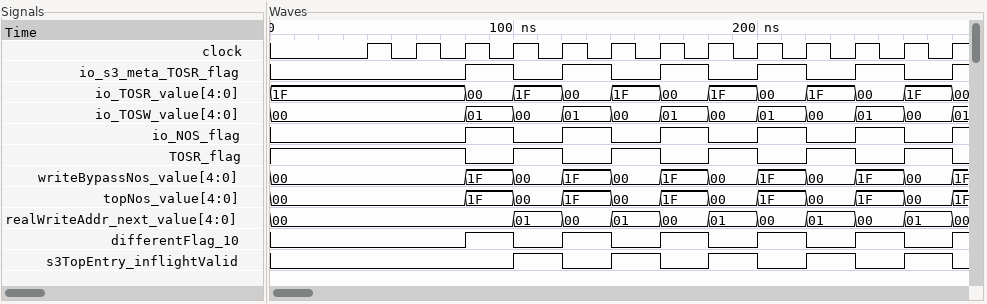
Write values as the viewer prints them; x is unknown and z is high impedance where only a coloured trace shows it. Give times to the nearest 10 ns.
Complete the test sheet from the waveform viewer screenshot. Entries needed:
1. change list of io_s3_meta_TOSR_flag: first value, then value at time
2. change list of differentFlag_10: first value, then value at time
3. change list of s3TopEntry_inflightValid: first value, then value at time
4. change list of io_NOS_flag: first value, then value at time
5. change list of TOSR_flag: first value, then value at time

0, 1 at 80 ns, 0 at 100 ns, 1 at 120 ns, 0 at 140 ns, 1 at 160 ns, 0 at 180 ns, 1 at 200 ns, 0 at 220 ns, 1 at 240 ns, 0 at 260 ns, 1 at 280 ns
0, 1 at 80 ns, 0 at 100 ns, 1 at 120 ns, 0 at 140 ns, 1 at 160 ns, 0 at 180 ns, 1 at 200 ns, 0 at 220 ns, 1 at 240 ns, 0 at 260 ns, 1 at 280 ns
0, 1 at 100 ns, 0 at 120 ns, 1 at 140 ns, 0 at 160 ns, 1 at 180 ns, 0 at 200 ns, 1 at 220 ns, 0 at 240 ns, 1 at 260 ns, 0 at 280 ns
0, 1 at 80 ns, 0 at 100 ns, 1 at 120 ns, 0 at 140 ns, 1 at 160 ns, 0 at 180 ns, 1 at 200 ns, 0 at 220 ns, 1 at 240 ns, 0 at 260 ns, 1 at 280 ns
1, 0 at 80 ns, 1 at 100 ns, 0 at 120 ns, 1 at 140 ns, 0 at 160 ns, 1 at 180 ns, 0 at 200 ns, 1 at 220 ns, 0 at 240 ns, 1 at 260 ns, 0 at 280 ns
